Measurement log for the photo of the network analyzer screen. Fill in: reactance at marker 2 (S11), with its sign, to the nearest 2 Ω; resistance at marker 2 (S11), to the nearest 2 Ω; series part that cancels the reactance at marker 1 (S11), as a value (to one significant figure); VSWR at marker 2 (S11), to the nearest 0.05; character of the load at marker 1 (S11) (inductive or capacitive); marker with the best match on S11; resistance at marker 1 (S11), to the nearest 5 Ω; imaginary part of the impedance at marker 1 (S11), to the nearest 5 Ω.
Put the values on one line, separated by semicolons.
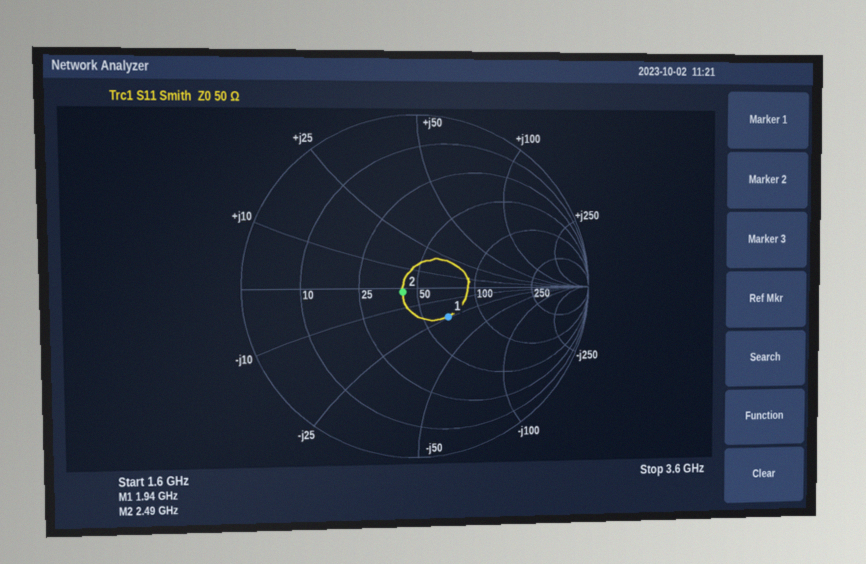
-2 Ω; 42 Ω; 2 nH; 1.20; capacitive; marker 2; 65 Ω; -25 Ω
